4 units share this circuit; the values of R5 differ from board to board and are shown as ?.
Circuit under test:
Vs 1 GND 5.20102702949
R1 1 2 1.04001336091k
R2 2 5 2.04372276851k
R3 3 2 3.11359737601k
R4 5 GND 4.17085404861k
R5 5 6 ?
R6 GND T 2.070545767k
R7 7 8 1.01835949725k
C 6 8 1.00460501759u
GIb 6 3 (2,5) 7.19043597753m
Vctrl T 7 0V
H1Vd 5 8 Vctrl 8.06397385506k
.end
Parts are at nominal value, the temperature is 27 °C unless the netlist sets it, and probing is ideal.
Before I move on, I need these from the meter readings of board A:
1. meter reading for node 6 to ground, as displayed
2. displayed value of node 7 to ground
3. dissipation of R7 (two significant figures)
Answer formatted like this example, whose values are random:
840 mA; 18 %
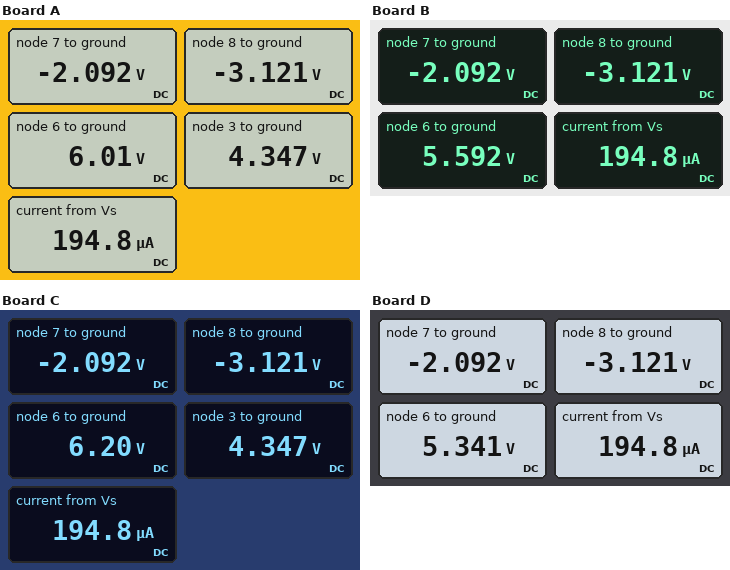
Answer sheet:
6.01 V; -2.092 V; 1.0 mW
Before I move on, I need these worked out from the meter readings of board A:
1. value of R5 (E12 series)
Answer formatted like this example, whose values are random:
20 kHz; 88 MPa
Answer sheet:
4.7 kΩ
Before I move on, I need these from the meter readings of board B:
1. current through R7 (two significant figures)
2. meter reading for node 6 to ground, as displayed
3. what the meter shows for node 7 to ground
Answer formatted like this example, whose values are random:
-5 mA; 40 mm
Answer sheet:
1.0 mA; 5.592 V; -2.092 V
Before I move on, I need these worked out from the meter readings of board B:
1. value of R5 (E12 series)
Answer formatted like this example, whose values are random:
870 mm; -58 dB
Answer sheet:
2.7 kΩ
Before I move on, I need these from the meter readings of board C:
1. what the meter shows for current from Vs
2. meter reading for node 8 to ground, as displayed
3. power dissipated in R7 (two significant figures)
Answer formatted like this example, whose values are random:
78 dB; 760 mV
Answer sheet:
194.8 µA; -3.121 V; 1.0 mW
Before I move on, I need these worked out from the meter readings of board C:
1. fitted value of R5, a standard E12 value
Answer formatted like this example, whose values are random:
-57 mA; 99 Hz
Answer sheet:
5.6 kΩ
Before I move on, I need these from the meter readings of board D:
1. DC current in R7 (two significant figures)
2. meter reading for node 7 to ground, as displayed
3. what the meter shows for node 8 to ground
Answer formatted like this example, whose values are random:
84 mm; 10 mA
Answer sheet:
1.0 mA; -2.092 V; -3.121 V
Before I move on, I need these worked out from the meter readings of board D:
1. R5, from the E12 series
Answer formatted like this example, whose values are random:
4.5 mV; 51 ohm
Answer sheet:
1.5 kΩ
